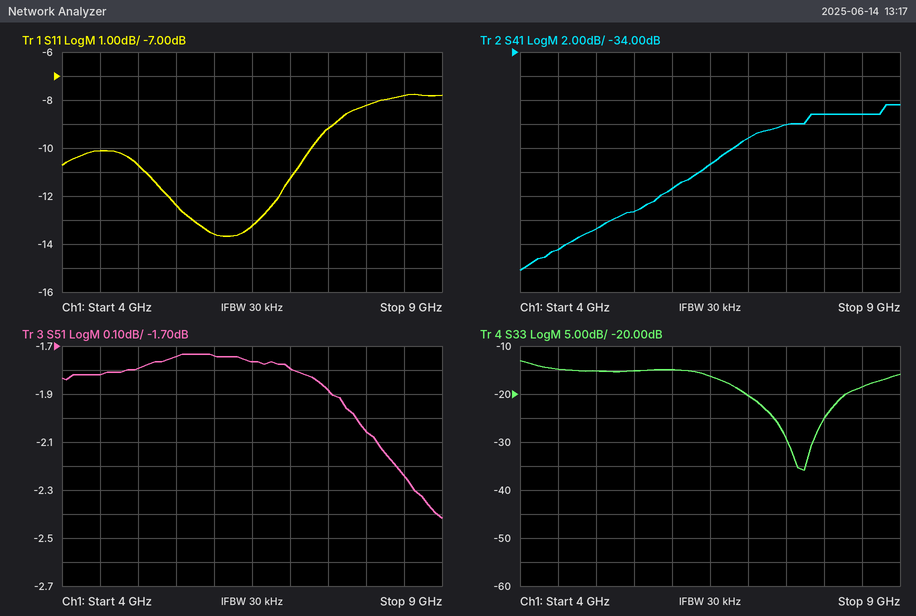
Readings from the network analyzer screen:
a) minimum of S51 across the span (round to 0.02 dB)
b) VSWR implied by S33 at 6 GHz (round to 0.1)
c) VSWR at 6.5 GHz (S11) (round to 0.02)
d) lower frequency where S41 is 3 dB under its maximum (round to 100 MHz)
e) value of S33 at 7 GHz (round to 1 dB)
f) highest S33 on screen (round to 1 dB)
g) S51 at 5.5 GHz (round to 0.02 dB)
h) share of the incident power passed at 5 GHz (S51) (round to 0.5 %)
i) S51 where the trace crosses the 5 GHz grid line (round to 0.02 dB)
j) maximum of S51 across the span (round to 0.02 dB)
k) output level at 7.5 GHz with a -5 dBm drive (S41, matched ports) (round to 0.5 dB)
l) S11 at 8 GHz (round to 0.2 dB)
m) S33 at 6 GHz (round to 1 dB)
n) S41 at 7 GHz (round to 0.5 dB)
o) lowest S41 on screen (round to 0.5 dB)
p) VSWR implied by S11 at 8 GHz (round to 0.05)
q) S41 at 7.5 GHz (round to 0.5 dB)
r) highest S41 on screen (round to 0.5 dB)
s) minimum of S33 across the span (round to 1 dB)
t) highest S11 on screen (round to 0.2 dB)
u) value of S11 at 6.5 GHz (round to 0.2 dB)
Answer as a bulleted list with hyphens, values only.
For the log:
- -2.42 dB
- 1.4
- 1.56
- 6.9 GHz
- -20 dB
- -13 dB
- -1.74 dB
- 66.0 %
- -1.80 dB
- -1.74 dB
- -45.0 dBm
- -8.2 dB
- -15 dB
- -41.0 dB
- -52.0 dB
- 2.25
- -40.0 dB
- -38.5 dB
- -36 dB
- -7.8 dB
- -13.2 dB
